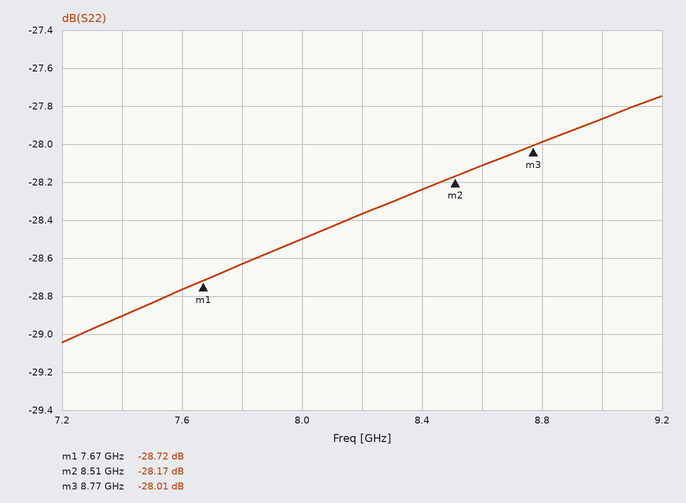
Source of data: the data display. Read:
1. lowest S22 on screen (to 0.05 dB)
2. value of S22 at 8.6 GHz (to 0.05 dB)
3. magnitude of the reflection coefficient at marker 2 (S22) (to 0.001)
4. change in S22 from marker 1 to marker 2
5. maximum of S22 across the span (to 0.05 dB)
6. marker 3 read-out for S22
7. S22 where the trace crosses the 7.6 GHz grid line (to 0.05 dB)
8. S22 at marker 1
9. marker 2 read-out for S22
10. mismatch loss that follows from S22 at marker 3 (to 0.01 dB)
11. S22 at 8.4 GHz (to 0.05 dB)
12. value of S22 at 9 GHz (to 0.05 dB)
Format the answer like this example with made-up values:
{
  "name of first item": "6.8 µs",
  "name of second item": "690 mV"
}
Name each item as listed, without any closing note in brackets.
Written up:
{
  "lowest S22 on screen": "-29.05 dB",
  "value of S22 at 8.6 GHz": "-28.10 dB",
  "magnitude of the reflection coefficient at marker 2 (S22)": "0.039",
  "change in S22 from marker 1 to marker 2": "0.55 dB",
  "maximum of S22 across the span": "-27.75 dB",
  "marker 3 read-out for S22": "-28.01 dB",
  "S22 where the trace crosses the 7.6 GHz grid line": "-28.75 dB",
  "S22 at marker 1": "-28.72 dB",
  "marker 2 read-out for S22": "-28.17 dB",
  "mismatch loss that follows from S22 at marker 3": "0.01 dB",
  "S22 at 8.4 GHz": "-28.25 dB",
  "value of S22 at 9 GHz": "-27.85 dB"
}
